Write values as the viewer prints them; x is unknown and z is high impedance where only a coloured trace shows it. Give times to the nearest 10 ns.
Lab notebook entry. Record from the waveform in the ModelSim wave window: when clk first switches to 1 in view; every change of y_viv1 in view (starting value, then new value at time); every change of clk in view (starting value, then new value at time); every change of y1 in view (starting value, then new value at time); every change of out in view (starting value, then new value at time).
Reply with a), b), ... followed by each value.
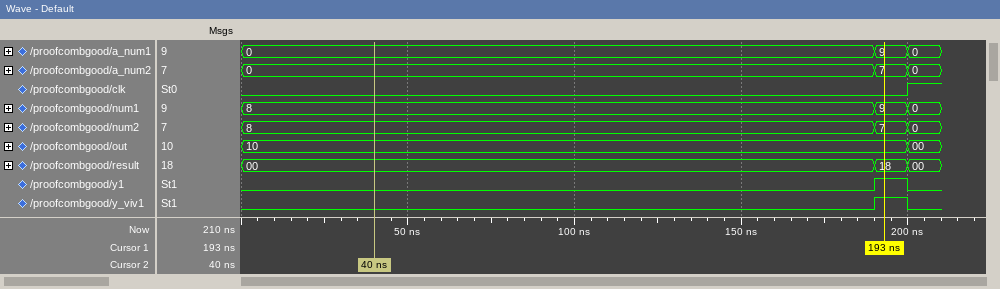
a) 200 ns
b) 0, 1 at 190 ns, 0 at 200 ns
c) 0, 1 at 200 ns
d) 0, 1 at 190 ns, 0 at 200 ns
e) 10, 00 at 200 ns
